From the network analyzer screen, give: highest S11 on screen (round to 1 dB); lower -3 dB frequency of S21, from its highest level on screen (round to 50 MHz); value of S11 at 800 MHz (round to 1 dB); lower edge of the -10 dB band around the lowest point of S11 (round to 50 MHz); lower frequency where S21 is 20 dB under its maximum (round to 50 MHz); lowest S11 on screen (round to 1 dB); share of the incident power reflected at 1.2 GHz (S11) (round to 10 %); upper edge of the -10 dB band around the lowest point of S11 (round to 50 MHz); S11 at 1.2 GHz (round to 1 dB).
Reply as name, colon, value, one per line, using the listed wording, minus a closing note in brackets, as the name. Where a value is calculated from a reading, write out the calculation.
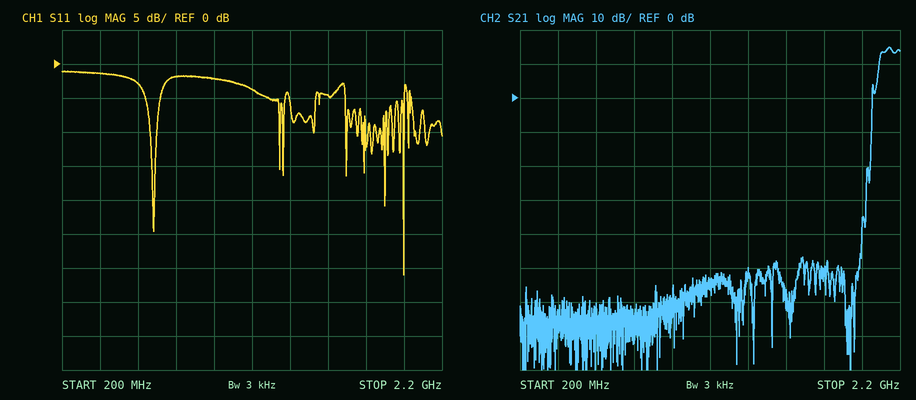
highest S11 on screen: -1 dB
lower -3 dB frequency of S21, from its highest level on screen: 2.10 GHz
value of S11 at 800 MHz: -2 dB
lower edge of the -10 dB band around the lowest point of S11: 2.00 GHz
lower frequency where S21 is 20 dB under its maximum: 2.05 GHz
lowest S11 on screen: -31 dB
share of the incident power reflected at 1.2 GHz (S11): 10^(-4/10) ≈ 40 %
upper edge of the -10 dB band around the lowest point of S11: 2.00 GHz
S11 at 1.2 GHz: -4 dB
